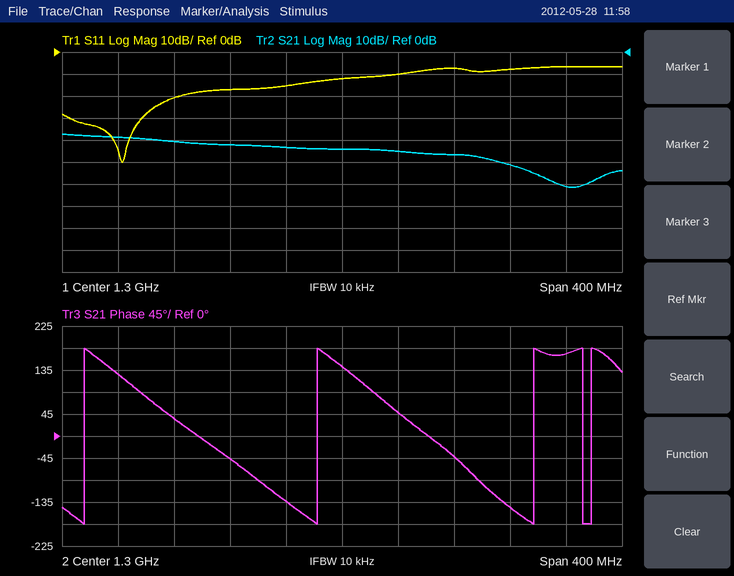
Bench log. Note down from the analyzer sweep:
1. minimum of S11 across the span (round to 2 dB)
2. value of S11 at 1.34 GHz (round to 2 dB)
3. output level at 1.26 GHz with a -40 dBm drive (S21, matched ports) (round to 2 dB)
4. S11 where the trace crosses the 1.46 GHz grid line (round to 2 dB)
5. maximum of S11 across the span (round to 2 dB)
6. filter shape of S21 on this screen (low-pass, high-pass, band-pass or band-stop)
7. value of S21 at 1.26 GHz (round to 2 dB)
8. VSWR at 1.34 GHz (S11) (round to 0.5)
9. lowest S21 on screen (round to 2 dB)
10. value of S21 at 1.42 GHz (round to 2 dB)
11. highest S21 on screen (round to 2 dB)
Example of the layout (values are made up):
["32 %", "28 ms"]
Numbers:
["-50 dB", "-10 dB", "-84 dBm", "-6 dB", "-6 dB", "low-pass", "-44 dB", "2.0", "-62 dB", "-52 dB", "-38 dB"]
